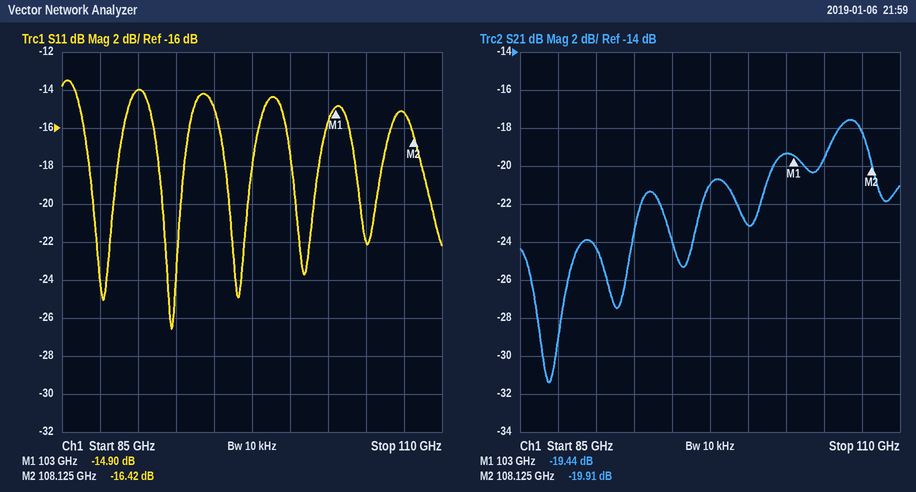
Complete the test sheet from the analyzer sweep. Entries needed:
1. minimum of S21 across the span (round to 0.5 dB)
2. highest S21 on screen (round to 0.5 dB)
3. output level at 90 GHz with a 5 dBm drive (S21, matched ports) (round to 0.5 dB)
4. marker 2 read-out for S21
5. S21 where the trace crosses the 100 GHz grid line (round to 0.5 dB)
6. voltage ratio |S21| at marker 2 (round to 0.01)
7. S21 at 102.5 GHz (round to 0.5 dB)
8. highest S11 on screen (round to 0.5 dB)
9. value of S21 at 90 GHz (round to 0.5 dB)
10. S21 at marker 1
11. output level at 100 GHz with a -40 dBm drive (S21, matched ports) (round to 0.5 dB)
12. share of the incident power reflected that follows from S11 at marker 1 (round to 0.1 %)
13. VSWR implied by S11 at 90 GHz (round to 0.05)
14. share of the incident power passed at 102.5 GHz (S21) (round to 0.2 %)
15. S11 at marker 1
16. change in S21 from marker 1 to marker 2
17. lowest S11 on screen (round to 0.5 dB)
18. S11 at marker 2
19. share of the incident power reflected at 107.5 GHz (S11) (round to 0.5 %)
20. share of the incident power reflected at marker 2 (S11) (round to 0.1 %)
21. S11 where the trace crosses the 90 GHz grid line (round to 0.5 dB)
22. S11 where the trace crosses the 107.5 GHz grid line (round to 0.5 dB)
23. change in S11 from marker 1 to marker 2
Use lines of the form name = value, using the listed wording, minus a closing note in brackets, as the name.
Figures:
minimum of S21 across the span = -31.5 dB
highest S21 on screen = -17.5 dB
output level at 90 GHz with a 5 dBm drive (S21, matched ports) = -19.5 dBm
marker 2 read-out for S21 = -19.91 dB
S21 where the trace crosses the 100 GHz grid line = -23.0 dB
voltage ratio |S21| at marker 2 = 0.10
S21 at 102.5 GHz = -19.5 dB
highest S11 on screen = -13.5 dB
value of S21 at 90 GHz = -24.5 dB
S21 at marker 1 = -19.44 dB
output level at 100 GHz with a -40 dBm drive (S21, matched ports) = -63.0 dBm
share of the incident power reflected that follows from S11 at marker 1 = 3.2 %
VSWR implied by S11 at 90 GHz = 1.50
share of the incident power passed at 102.5 GHz (S21) = 1.2 %
S11 at marker 1 = -14.90 dB
change in S21 from marker 1 to marker 2 = -0.47 dB
lowest S11 on screen = -26.5 dB
S11 at marker 2 = -16.42 dB
share of the incident power reflected at 107.5 GHz (S11) = 3.0 %
share of the incident power reflected at marker 2 (S11) = 2.3 %
S11 where the trace crosses the 90 GHz grid line = -14.0 dB
S11 where the trace crosses the 107.5 GHz grid line = -15.0 dB
change in S11 from marker 1 to marker 2 = -1.52 dB
